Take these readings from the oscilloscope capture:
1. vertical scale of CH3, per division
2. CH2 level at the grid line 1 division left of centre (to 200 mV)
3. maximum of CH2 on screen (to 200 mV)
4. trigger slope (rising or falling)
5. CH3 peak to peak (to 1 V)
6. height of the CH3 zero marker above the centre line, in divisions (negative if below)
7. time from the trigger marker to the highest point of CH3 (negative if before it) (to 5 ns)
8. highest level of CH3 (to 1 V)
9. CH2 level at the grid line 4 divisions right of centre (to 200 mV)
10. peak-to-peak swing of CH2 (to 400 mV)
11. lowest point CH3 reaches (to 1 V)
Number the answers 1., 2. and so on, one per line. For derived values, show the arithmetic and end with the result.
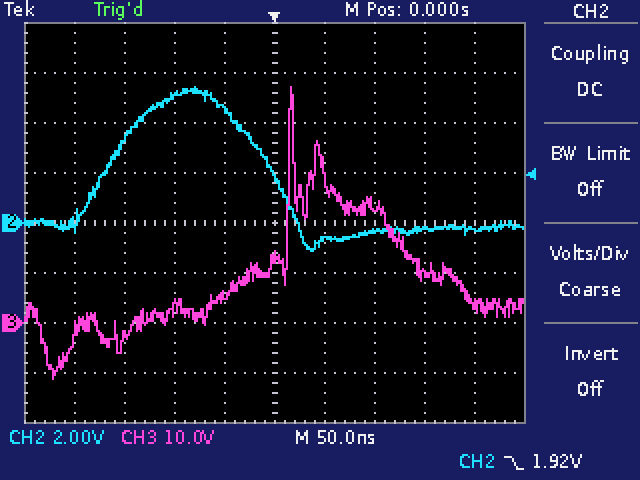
1. 10 V
2. 4.6 V
3. 5.4 V
4. falling
5. 47 V − (-11 V) = 58 V
6. -2.0 div
7. +15 ns
8. 47 V
9. -200 mV
10. 6.4 V
11. -11 V
